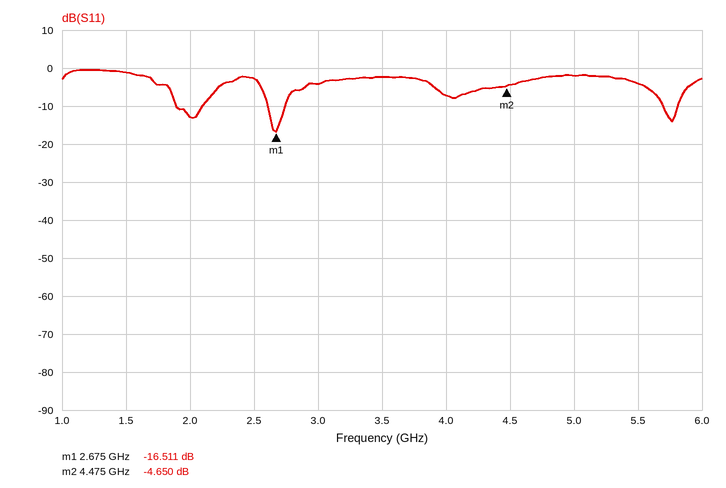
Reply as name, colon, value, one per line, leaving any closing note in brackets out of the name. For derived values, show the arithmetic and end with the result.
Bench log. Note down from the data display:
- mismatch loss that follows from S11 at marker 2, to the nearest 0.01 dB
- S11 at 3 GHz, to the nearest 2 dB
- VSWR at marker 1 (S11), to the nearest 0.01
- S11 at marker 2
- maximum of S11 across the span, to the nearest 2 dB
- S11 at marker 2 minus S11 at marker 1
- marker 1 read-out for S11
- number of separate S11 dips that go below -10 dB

mismatch loss that follows from S11 at marker 2, to the nearest 0.01 dB: −10 log10(1 − 10^(-4.65/10)) ≈ 1.82 dB
S11 at 3 GHz, to the nearest 2 dB: -4 dB
VSWR at marker 1 (S11), to the nearest 0.01: (1 + 0.1494)/(1 − 0.1494) ≈ 1.35
S11 at marker 2: -4.650 dB
maximum of S11 across the span, to the nearest 2 dB: 0 dB
S11 at marker 2 minus S11 at marker 1: -4.65 − (-16.511) = 11.861 dB
marker 1 read-out for S11: -16.511 dB
number of separate S11 dips that go below -10 dB: 3
